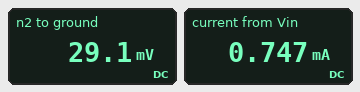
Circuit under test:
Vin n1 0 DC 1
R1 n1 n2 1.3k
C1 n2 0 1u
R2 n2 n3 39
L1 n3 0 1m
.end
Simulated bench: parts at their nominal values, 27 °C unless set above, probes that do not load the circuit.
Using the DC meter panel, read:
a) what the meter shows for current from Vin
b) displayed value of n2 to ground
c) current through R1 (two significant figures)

0.747 mA
29.1 mV
750 µA
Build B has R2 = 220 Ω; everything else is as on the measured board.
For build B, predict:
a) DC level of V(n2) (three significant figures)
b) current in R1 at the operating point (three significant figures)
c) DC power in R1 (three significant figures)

145 mV
658 µA
563 µW
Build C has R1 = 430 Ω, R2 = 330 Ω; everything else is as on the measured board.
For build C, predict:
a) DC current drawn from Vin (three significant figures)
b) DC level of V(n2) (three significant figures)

1.32 mA
434 mV
